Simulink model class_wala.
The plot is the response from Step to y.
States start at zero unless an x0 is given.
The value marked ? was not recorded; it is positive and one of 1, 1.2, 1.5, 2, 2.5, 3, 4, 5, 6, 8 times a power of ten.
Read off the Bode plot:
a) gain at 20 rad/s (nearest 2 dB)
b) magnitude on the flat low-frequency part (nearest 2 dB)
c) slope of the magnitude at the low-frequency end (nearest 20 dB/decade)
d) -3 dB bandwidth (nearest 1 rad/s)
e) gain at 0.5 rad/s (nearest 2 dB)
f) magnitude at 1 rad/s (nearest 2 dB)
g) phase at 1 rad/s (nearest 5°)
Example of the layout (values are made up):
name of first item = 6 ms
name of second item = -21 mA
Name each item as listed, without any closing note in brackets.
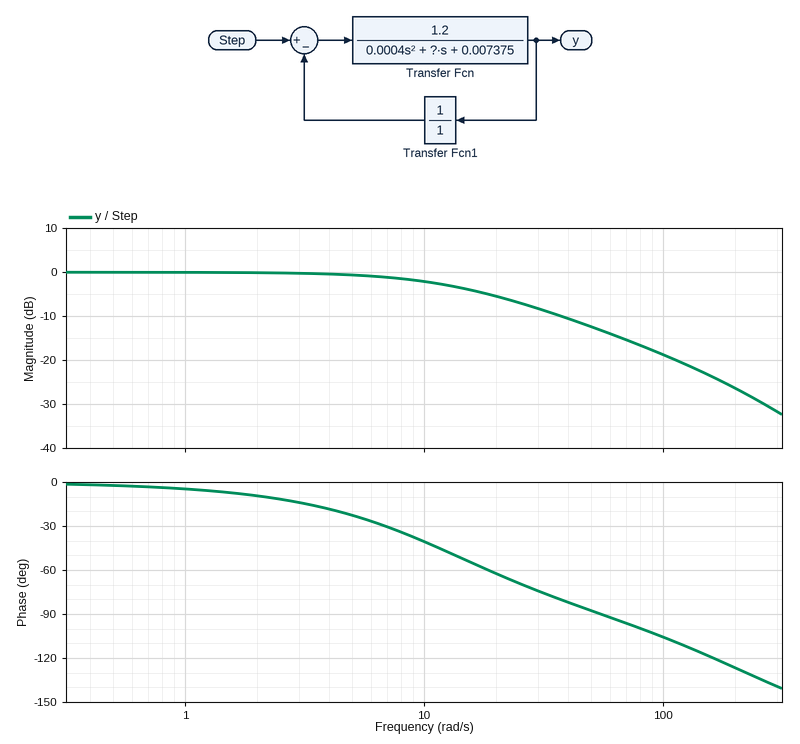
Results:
gain at 20 rad/s = -6 dB
magnitude on the flat low-frequency part = 0 dB
slope of the magnitude at the low-frequency end = 0 dB/decade
-3 dB bandwidth = 13 rad/s
gain at 0.5 rad/s = 0 dB
magnitude at 1 rad/s = 0 dB
phase at 1 rad/s = -5°
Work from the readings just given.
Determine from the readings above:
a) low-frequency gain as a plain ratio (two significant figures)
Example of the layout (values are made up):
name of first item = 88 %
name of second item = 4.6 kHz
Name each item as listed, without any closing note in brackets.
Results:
low-frequency gain as a plain ratio = 1.0
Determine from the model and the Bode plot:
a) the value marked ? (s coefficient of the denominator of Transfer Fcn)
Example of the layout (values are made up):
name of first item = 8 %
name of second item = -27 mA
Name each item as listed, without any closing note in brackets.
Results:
the value marked ? = 0.1
